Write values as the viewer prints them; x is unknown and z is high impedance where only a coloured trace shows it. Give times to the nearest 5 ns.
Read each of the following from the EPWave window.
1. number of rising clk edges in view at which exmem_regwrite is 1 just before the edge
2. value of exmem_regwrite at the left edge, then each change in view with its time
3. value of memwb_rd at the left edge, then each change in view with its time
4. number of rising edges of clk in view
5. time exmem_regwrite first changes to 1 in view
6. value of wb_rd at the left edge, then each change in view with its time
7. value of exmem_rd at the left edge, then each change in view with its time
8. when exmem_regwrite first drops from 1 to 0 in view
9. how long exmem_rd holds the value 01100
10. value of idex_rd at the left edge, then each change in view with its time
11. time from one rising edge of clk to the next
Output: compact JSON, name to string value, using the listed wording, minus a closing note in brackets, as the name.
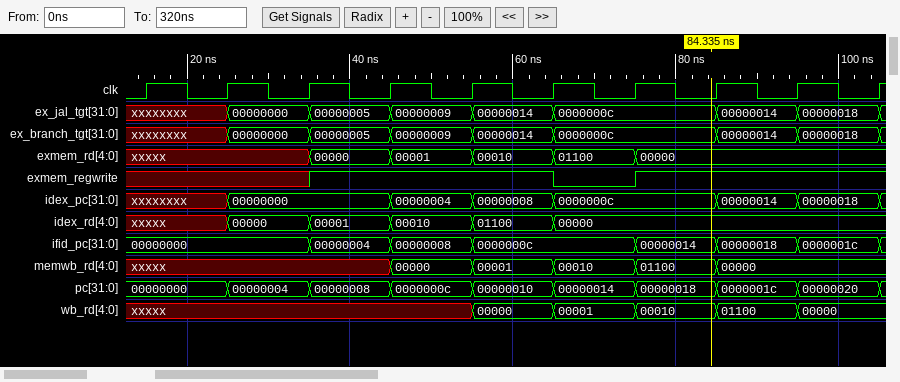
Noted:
{"number of rising clk edges in view at which exmem_regwrite is 1 just before the edge": "6", "value of exmem_regwrite at the left edge, then each change in view with its time": "x, 1 at 35 ns, 0 at 65 ns, 1 at 75 ns", "value of memwb_rd at the left edge, then each change in view with its time": "xxxxx, 00000 at 45 ns, 00001 at 55 ns, 00010 at 65 ns, 01100 at 75 ns, 00000 at 85 ns", "number of rising edges of clk in view": "10", "time exmem_regwrite first changes to 1 in view": "35 ns", "value of wb_rd at the left edge, then each change in view with its time": "xxxxx, 00000 at 55 ns, 00001 at 65 ns, 00010 at 75 ns, 01100 at 85 ns, 00000 at 95 ns", "value of exmem_rd at the left edge, then each change in view with its time": "xxxxx, 00000 at 35 ns, 00001 at 45 ns, 00010 at 55 ns, 01100 at 65 ns, 00000 at 75 ns", "when exmem_regwrite first drops from 1 to 0 in view": "65 ns", "how long exmem_rd holds the value 01100": "10 ns", "value of idex_rd at the left edge, then each change in view with its time": "xxxxx, 00000 at 25 ns, 00001 at 35 ns, 00010 at 45 ns, 01100 at 55 ns, 00000 at 65 ns", "time from one rising edge of clk to the next": "10 ns"}
